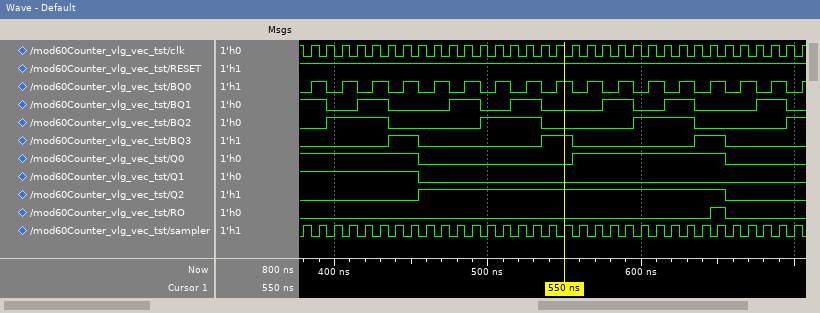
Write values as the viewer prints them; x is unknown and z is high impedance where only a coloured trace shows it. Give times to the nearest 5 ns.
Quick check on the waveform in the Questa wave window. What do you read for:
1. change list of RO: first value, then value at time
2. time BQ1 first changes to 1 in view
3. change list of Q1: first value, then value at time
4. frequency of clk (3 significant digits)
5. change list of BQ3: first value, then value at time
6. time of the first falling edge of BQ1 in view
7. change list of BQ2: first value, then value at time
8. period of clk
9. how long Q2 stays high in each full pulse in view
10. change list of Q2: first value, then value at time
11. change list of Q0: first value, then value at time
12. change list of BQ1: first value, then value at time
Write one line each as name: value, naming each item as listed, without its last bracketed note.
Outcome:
change list of RO: first value, then value at time: 0, 1 at 645 ns, 0 at 655 ns
time BQ1 first changes to 1 in view: 415 ns
change list of Q1: first value, then value at time: 1, 0 at 455 ns
frequency of clk: 100 MHz
change list of BQ3: first value, then value at time: 0, 1 at 435 ns, 0 at 455 ns, 1 at 535 ns, 0 at 555 ns, 1 at 635 ns, 0 at 655 ns
time of the first falling edge of BQ1 in view: 395 ns
change list of BQ2: first value, then value at time: 0, 1 at 395 ns, 0 at 435 ns, 1 at 495 ns, 0 at 535 ns, 1 at 595 ns, 0 at 635 ns, 1 at 695 ns
period of clk: 10 ns
how long Q2 stays high in each full pulse in view: 200 ns
change list of Q2: first value, then value at time: 0, 1 at 455 ns, 0 at 655 ns
change list of Q0: first value, then value at time: 1, 0 at 455 ns, 1 at 555 ns, 0 at 655 ns
change list of BQ1: first value, then value at time: 1, 0 at 395 ns, 1 at 415 ns, 0 at 435 ns, 1 at 475 ns, 0 at 495 ns, 1 at 515 ns, 0 at 535 ns, 1 at 575 ns, 0 at 595 ns, 1 at 615 ns, 0 at 635 ns, 1 at 675 ns, 0 at 695 ns
